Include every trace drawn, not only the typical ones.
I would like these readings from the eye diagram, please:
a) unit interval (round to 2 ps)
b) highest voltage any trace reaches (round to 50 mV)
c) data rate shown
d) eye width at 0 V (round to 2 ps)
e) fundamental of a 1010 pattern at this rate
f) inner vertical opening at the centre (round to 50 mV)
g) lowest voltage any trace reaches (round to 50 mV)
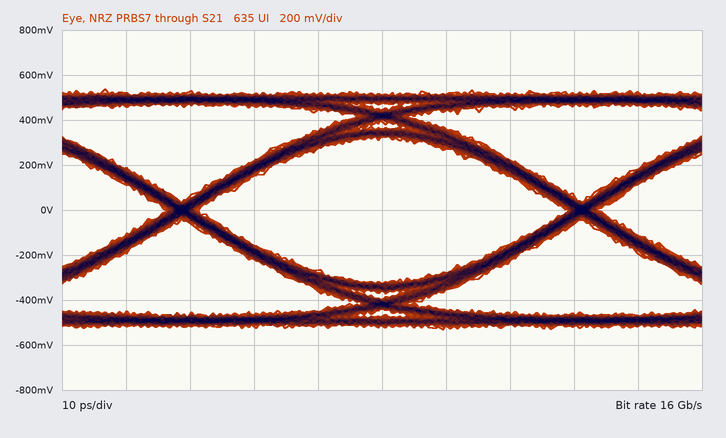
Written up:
62 ps
550 mV
16 Gb/s
58 ps
8 GHz
650 mV
-550 mV
